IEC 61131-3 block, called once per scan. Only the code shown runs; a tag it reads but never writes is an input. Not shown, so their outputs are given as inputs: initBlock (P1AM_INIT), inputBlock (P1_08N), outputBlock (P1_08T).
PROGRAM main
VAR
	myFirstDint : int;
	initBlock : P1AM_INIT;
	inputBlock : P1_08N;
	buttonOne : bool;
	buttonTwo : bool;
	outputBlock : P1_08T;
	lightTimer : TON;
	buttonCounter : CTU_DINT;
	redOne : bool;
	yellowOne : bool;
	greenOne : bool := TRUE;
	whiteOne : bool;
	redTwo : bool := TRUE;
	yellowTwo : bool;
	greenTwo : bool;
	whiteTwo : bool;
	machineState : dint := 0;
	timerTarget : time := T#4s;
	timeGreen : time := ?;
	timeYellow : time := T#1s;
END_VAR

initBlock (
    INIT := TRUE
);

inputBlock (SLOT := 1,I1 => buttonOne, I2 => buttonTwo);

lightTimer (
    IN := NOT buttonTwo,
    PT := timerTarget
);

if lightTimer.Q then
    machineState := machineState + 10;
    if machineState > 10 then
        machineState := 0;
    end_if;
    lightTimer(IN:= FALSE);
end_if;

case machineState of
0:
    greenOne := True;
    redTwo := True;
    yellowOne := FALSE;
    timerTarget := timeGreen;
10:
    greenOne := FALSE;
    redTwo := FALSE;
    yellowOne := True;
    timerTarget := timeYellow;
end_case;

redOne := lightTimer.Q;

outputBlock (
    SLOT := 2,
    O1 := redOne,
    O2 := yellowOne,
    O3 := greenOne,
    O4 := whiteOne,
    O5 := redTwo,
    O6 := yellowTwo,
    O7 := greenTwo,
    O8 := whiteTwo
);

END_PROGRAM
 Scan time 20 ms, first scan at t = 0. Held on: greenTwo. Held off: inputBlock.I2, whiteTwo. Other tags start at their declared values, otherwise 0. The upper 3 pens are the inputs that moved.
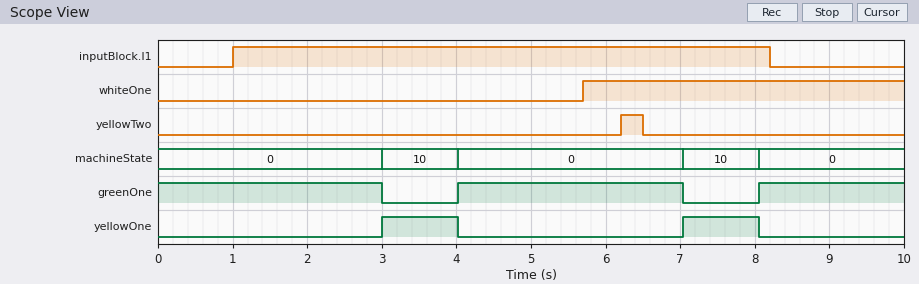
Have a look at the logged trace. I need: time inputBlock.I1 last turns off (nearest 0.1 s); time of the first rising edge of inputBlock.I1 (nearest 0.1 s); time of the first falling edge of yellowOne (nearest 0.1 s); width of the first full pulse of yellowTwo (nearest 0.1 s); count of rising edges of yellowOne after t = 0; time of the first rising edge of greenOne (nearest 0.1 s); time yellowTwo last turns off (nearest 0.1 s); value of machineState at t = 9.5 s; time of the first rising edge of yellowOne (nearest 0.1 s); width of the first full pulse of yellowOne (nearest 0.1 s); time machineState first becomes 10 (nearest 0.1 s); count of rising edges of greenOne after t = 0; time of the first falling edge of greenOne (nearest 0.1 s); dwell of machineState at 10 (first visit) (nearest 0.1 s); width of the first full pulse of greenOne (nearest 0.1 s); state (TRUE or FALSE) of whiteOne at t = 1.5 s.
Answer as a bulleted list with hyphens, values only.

- 8.2 s
- 1.0 s
- 4.0 s
- 0.3 s
- 2
- 4.0 s
- 6.5 s
- 0
- 3.0 s
- 1.0 s
- 3.0 s
- 2
- 3.0 s
- 1.0 s
- 3.0 s
- FALSE
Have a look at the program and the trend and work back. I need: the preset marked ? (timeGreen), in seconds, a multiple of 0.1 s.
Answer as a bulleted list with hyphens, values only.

- 3.0 s
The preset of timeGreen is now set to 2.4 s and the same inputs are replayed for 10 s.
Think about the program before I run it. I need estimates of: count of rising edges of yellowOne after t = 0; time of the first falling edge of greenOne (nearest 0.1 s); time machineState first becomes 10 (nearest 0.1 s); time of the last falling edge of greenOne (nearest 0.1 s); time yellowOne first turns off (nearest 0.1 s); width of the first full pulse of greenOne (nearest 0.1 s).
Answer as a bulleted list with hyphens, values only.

- 3
- 2.4 s
- 2.4 s
- 9.3 s
- 3.4 s
- 2.4 s
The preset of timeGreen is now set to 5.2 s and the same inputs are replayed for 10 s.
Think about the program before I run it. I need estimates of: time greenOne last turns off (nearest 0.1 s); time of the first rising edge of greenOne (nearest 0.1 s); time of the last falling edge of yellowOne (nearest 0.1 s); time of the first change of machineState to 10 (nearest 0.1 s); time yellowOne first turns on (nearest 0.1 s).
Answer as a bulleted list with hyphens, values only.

- 5.2 s
- 6.2 s
- 6.2 s
- 5.2 s
- 5.2 s
